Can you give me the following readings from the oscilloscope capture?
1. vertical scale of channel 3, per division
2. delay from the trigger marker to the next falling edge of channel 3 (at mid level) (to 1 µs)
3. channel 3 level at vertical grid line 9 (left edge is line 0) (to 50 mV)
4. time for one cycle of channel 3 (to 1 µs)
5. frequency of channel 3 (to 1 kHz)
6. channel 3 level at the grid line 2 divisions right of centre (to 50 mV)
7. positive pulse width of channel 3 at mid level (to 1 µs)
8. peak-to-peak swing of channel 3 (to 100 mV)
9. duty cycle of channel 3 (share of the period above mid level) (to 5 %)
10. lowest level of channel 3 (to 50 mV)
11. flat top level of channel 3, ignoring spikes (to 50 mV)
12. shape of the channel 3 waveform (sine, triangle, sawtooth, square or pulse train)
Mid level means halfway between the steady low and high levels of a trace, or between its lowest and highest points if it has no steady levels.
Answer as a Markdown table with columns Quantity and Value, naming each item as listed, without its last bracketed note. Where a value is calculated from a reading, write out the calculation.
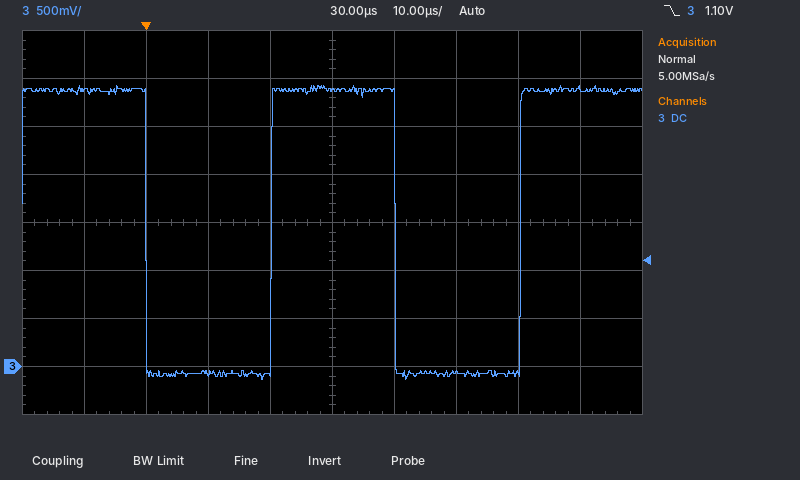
| Quantity | Value |
|---|---|
| vertical scale of channel 3, per division | 500 mV |
| delay from the trigger marker to the next falling edge of channel 3 (at mid level) | 40 µs |
| channel 3 level at vertical grid line 9 (left edge is line 0) | 2.90 V |
| time for one cycle of channel 3 | 40 µs |
| frequency of channel 3 | 1 / 40 µs ≈ 25 kHz |
| channel 3 level at the grid line 2 divisions right of centre | -50 mV |
| positive pulse width of channel 3 at mid level | 20 µs |
| peak-to-peak swing of channel 3 | 3.10 V |
| duty cycle of channel 3 (share of the period above mid level) | 20 µs / 40 µs ≈ 50 % |
| lowest level of channel 3 | -150 mV |
| flat top level of channel 3, ignoring spikes | 2.90 V |
| shape of the channel 3 waveform | square |
